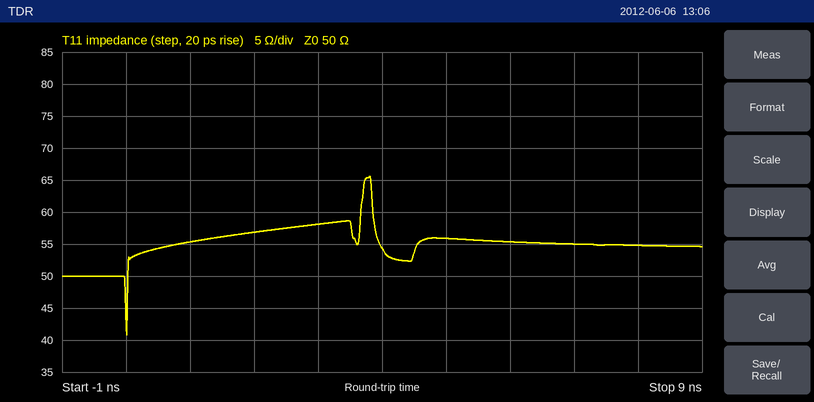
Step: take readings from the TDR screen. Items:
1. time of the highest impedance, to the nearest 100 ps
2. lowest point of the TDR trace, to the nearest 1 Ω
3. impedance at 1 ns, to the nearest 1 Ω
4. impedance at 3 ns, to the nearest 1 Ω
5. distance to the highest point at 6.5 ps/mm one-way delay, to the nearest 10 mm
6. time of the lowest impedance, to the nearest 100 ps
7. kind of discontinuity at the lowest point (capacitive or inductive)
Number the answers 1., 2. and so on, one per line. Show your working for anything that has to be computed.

1. 3.8 ns
2. 41 Ω
3. 55 Ω
4. 58 Ω
5. 3.8 ns / 2 / 6.5 ps/mm ≈ 292 mm, so 290 mm to the nearest 10 mm
6. 0.0 ns
7. capacitive
